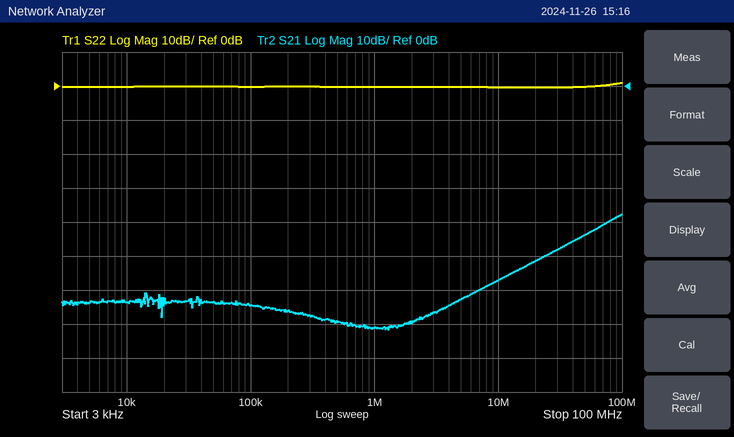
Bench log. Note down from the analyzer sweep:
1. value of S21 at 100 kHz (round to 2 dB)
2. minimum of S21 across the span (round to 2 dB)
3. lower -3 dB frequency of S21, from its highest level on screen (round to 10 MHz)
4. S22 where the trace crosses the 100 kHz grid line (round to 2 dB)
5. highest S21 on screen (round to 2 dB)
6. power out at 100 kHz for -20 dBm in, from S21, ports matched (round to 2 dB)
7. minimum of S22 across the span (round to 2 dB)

-64 dB
-72 dB
70 MHz
0 dB
-38 dB
-84 dBm
0 dB
